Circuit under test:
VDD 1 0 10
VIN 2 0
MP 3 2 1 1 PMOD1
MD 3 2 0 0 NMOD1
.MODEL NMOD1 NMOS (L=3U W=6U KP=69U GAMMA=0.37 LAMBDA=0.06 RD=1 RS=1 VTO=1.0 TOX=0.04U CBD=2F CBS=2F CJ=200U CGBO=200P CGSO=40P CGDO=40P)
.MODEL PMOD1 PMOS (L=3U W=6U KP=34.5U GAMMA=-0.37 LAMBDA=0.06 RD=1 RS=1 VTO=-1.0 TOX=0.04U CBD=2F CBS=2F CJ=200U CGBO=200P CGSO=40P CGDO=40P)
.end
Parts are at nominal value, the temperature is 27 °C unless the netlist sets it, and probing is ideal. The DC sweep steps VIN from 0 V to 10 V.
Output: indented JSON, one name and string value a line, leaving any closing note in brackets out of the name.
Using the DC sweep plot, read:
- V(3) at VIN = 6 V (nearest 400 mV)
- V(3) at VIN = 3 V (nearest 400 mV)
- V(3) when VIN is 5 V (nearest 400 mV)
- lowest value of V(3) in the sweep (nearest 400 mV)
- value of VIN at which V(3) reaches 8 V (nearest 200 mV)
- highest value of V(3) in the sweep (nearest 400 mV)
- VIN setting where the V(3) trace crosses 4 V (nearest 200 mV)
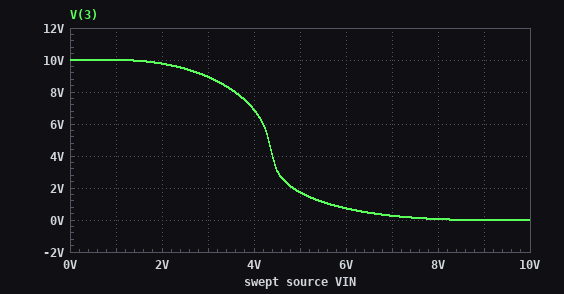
{
  "V(3) at VIN = 6 V": "800 mV",
  "V(3) at VIN = 3 V": "8.8 V",
  "V(3) when VIN is 5 V": "1.6 V",
  "lowest value of V(3) in the sweep": "0 V",
  "value of VIN at which V(3) reaches 8 V": "3.6 V",
  "highest value of V(3) in the sweep": "10.0 V",
  "VIN setting where the V(3) trace crosses 4 V": "4.4 V"
}
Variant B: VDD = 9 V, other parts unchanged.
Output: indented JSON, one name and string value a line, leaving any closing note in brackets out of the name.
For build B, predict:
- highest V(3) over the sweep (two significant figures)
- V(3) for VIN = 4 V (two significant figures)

{
  "highest V(3) over the sweep": "9.0 V",
  "V(3) for VIN = 4 V": "3.3 V"
}
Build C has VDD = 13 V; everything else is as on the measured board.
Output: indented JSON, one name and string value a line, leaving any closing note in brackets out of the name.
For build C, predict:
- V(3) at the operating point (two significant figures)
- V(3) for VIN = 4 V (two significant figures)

{
  "V(3) at the operating point": "13 V",
  "V(3) for VIN = 4 V": "11 V"
}
